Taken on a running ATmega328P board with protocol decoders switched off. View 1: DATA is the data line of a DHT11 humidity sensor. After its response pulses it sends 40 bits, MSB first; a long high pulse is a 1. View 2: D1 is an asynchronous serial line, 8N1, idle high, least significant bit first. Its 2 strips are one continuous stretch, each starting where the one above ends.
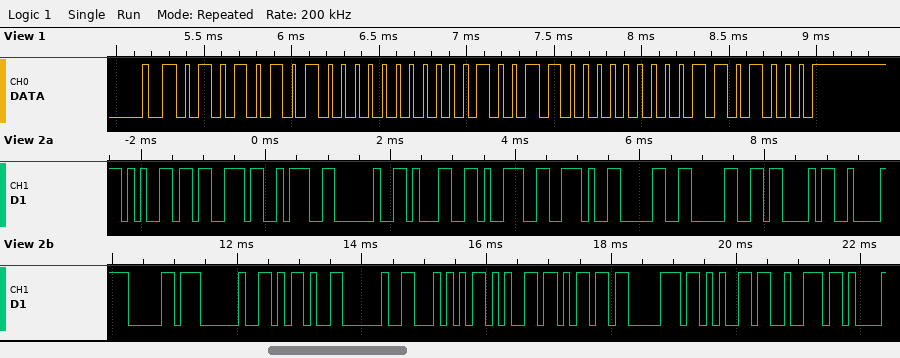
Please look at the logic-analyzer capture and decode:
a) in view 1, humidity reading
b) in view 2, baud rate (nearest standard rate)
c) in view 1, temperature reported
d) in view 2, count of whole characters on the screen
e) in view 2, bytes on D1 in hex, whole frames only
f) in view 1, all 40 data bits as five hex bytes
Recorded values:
85 %
9600 baud
19.0 °C
21
65 73 3A 20 31 39 2E 30 30 43 C2 B0 20 2D 20 54 65 6D 70 65 72
55 00 13 00 68
